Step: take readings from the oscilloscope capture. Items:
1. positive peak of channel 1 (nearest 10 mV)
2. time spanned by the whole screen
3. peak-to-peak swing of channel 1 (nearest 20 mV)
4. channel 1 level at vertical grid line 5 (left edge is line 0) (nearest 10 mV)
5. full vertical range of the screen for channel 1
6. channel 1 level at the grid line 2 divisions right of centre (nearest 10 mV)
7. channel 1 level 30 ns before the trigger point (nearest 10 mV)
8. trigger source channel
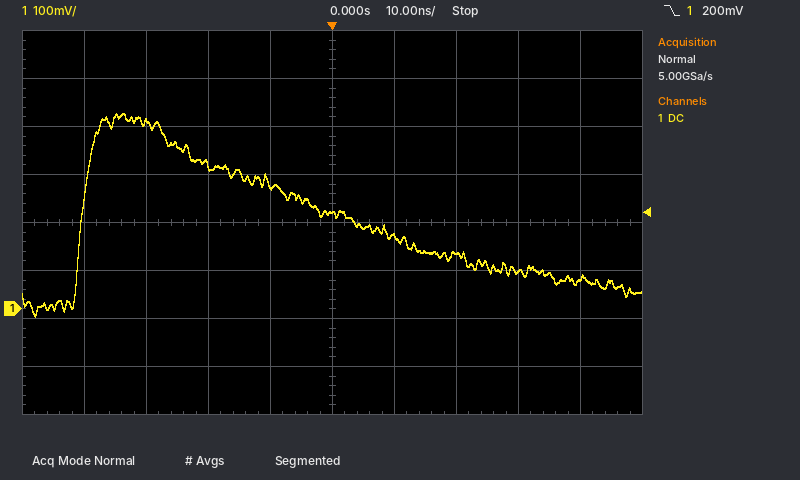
410 mV
100 ns
420 mV
200 mV
800 mV
120 mV
390 mV
channel 1
